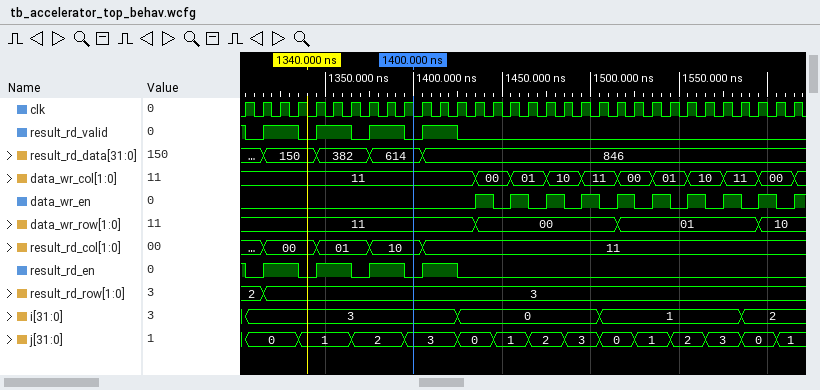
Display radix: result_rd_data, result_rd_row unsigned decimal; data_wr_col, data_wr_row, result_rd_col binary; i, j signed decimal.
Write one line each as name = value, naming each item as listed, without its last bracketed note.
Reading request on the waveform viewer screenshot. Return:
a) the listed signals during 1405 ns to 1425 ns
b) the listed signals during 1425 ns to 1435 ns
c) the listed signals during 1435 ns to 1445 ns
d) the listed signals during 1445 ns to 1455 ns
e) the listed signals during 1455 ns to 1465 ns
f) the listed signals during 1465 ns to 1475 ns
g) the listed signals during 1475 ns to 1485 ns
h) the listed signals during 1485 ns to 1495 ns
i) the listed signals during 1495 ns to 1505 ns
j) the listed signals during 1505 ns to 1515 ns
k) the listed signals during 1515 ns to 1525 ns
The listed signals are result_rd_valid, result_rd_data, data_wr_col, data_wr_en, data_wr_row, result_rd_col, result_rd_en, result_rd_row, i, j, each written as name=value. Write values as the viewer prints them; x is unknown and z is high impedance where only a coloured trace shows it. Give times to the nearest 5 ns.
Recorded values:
the listed signals during 1405 ns to 1425 ns = result_rd_valid=1, result_rd_data=846, data_wr_col=11, data_wr_en=0, data_wr_row=11, result_rd_col=11, result_rd_en=1, result_rd_row=3, i=3, j=3
the listed signals during 1425 ns to 1435 ns = result_rd_valid=0, result_rd_data=846, data_wr_col=11, data_wr_en=0, data_wr_row=11, result_rd_col=11, result_rd_en=0, result_rd_row=3, i=0, j=0
the listed signals during 1435 ns to 1445 ns = result_rd_valid=0, result_rd_data=846, data_wr_col=00, data_wr_en=1, data_wr_row=00, result_rd_col=11, result_rd_en=0, result_rd_row=3, i=0, j=0
the listed signals during 1445 ns to 1455 ns = result_rd_valid=0, result_rd_data=846, data_wr_col=00, data_wr_en=0, data_wr_row=00, result_rd_col=11, result_rd_en=0, result_rd_row=3, i=0, j=1
the listed signals during 1455 ns to 1465 ns = result_rd_valid=0, result_rd_data=846, data_wr_col=01, data_wr_en=1, data_wr_row=00, result_rd_col=11, result_rd_en=0, result_rd_row=3, i=0, j=1
the listed signals during 1465 ns to 1475 ns = result_rd_valid=0, result_rd_data=846, data_wr_col=01, data_wr_en=0, data_wr_row=00, result_rd_col=11, result_rd_en=0, result_rd_row=3, i=0, j=2
the listed signals during 1475 ns to 1485 ns = result_rd_valid=0, result_rd_data=846, data_wr_col=10, data_wr_en=1, data_wr_row=00, result_rd_col=11, result_rd_en=0, result_rd_row=3, i=0, j=2
the listed signals during 1485 ns to 1495 ns = result_rd_valid=0, result_rd_data=846, data_wr_col=10, data_wr_en=0, data_wr_row=00, result_rd_col=11, result_rd_en=0, result_rd_row=3, i=0, j=3
the listed signals during 1495 ns to 1505 ns = result_rd_valid=0, result_rd_data=846, data_wr_col=11, data_wr_en=1, data_wr_row=00, result_rd_col=11, result_rd_en=0, result_rd_row=3, i=0, j=3
the listed signals during 1505 ns to 1515 ns = result_rd_valid=0, result_rd_data=846, data_wr_col=11, data_wr_en=0, data_wr_row=00, result_rd_col=11, result_rd_en=0, result_rd_row=3, i=1, j=0
the listed signals during 1515 ns to 1525 ns = result_rd_valid=0, result_rd_data=846, data_wr_col=00, data_wr_en=1, data_wr_row=01, result_rd_col=11, result_rd_en=0, result_rd_row=3, i=1, j=0
